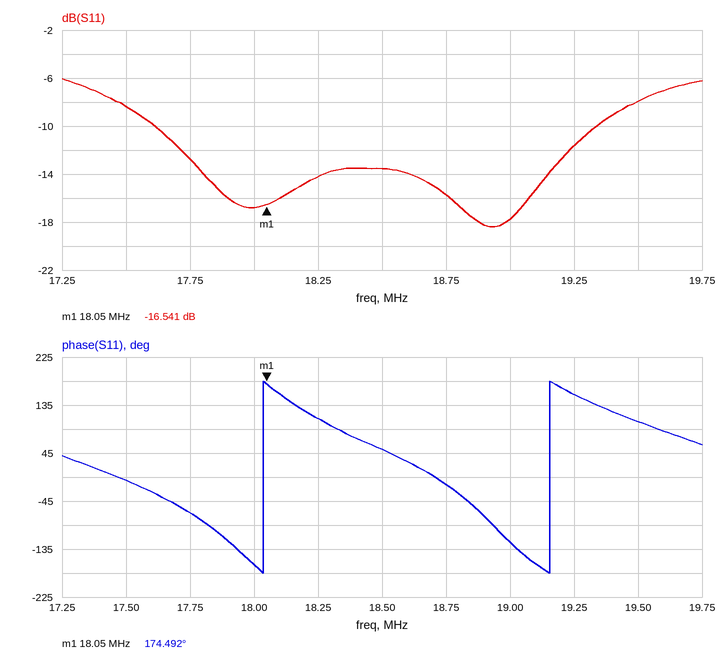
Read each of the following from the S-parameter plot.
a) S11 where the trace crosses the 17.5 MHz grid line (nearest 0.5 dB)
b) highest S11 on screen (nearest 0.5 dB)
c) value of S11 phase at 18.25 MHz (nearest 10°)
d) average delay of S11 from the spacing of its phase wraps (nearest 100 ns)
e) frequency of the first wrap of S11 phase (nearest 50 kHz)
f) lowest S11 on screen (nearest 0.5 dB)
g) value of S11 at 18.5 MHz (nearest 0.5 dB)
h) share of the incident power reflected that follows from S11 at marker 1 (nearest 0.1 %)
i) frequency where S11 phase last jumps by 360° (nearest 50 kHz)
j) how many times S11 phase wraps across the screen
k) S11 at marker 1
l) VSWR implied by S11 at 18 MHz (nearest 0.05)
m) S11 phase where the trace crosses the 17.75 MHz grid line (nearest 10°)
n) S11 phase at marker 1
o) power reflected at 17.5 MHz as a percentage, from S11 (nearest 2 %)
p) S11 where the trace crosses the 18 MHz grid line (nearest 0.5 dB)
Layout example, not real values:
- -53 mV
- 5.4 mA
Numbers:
- -8.5 dB
- -6.0 dB
- 110°
- 900 ns
- 18.05 MHz
- -18.5 dB
- -13.5 dB
- 2.2 %
- 19.15 MHz
- 2
- -16.541 dB
- 1.35
- -70°
- 174.492°
- 14 %
- -17.0 dB
